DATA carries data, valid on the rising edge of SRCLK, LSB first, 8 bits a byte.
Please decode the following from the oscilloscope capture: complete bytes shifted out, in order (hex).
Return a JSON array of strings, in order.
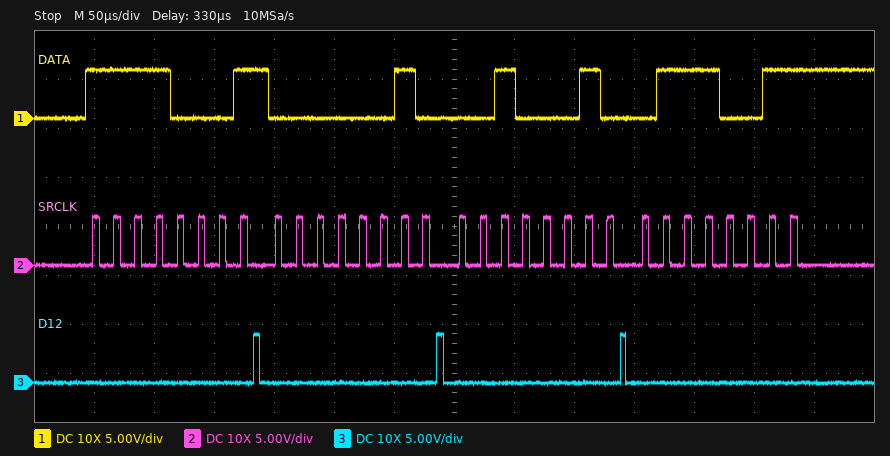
["0x8F 0x40 0x44 0xCE"]
